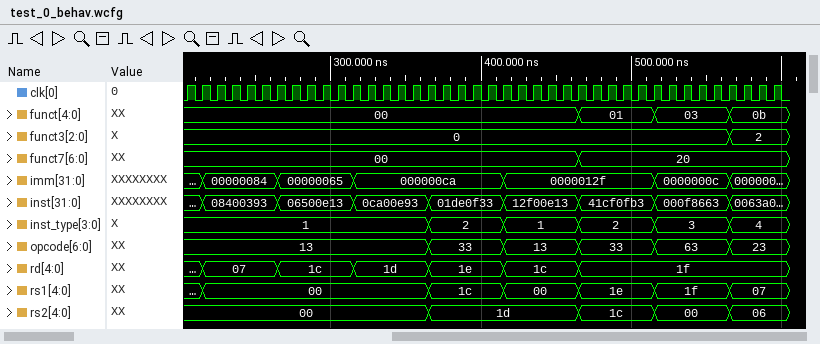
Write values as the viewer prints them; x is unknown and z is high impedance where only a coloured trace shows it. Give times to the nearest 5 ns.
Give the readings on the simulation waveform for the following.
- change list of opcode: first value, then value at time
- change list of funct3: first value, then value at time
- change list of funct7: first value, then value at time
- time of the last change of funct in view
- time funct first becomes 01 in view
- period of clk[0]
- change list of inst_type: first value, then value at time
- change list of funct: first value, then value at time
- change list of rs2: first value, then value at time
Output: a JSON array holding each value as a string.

["13, 33 at 365 ns, 13 at 415 ns, 33 at 465 ns, 63 at 515 ns, 23 at 565 ns", "0, 2 at 565 ns", "00, 20 at 465 ns", "565 ns", "465 ns", "10 ns", "1, 2 at 365 ns, 1 at 415 ns, 2 at 465 ns, 3 at 515 ns, 4 at 565 ns", "00, 01 at 465 ns, 03 at 515 ns, 0b at 565 ns", "00, 1d at 365 ns, 1c at 465 ns, 00 at 515 ns, 06 at 565 ns"]
